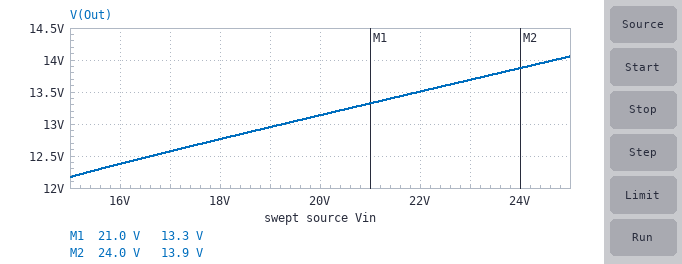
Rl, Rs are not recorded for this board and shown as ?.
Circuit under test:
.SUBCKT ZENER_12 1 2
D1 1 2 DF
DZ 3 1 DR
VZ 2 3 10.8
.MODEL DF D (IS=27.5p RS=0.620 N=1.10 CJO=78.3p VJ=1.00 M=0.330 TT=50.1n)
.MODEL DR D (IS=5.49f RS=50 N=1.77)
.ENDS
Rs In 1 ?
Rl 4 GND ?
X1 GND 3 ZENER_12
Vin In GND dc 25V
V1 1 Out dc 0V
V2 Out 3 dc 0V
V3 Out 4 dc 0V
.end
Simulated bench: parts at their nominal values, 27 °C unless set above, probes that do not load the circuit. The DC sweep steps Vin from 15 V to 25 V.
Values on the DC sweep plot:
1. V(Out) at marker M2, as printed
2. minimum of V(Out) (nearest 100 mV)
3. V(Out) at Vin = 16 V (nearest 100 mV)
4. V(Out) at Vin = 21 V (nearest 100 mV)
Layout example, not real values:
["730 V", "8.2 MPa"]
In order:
["13.9 V", "12.2 V", "12.4 V", "13.3 V"]
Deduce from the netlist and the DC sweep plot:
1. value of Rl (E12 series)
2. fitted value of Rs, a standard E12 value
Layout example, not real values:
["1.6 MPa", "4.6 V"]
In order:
["1.2 kΩ", "220 Ω"]
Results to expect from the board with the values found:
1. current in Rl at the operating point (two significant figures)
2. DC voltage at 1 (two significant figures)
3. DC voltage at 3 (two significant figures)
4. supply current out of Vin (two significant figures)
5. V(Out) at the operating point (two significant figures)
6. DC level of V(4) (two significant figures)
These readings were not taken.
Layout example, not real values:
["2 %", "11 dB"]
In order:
["12 mA", "14 V", "14 V", "50 mA", "14 V", "14 V"]
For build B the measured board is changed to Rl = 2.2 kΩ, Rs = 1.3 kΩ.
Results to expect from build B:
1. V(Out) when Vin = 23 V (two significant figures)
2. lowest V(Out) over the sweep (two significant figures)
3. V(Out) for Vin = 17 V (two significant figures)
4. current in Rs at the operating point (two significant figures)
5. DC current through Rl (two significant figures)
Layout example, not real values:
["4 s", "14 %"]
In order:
["12 V", "9.4 V", "11 V", "9.8 mA", "5.6 mA"]
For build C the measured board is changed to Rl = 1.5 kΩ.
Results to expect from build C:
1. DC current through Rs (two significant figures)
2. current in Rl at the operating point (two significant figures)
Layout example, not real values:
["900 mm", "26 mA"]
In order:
["49 mA", "9.4 mA"]
